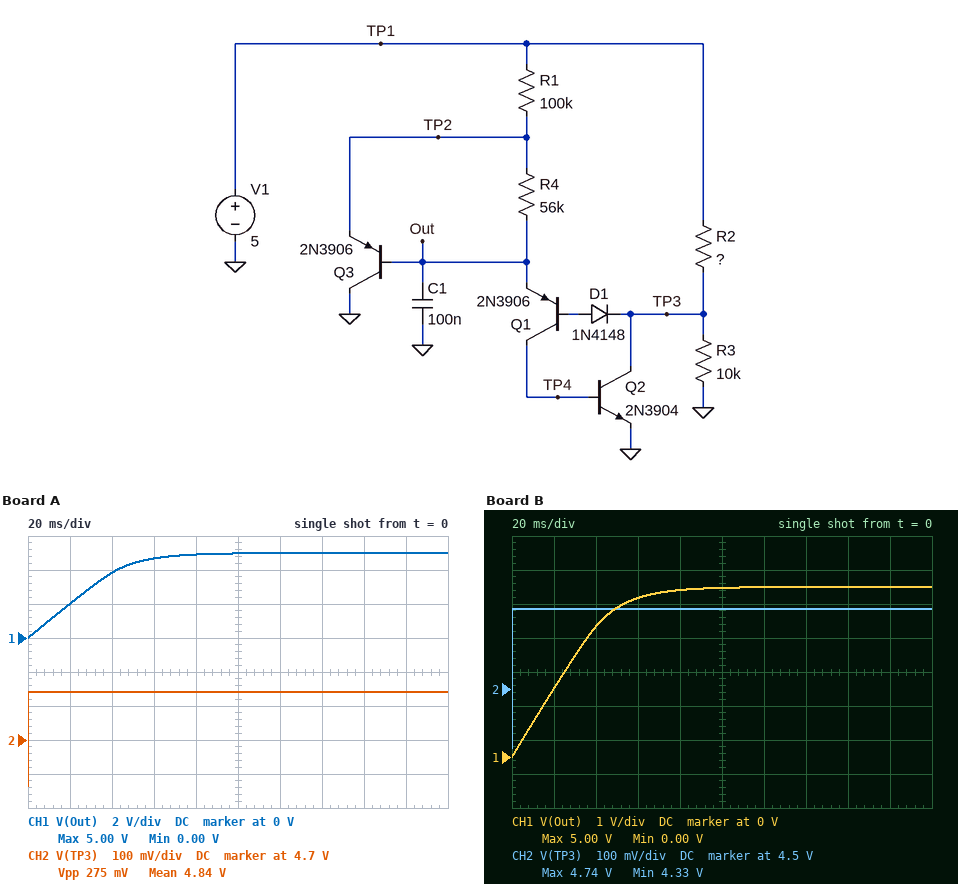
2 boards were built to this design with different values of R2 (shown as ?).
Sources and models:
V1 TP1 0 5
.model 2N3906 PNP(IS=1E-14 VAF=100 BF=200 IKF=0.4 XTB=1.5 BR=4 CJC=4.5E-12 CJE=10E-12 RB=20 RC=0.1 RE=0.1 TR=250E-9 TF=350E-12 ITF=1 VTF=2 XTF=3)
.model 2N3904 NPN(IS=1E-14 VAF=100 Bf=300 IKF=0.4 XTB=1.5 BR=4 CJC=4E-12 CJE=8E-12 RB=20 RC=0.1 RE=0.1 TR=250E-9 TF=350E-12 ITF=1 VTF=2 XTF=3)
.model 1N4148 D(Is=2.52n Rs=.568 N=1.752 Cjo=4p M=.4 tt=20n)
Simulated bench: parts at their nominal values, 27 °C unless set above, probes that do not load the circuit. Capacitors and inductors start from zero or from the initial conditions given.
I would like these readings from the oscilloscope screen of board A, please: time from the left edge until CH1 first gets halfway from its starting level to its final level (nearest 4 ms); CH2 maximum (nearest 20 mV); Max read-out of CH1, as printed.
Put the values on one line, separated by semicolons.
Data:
24 ms; 4.84 V; 5.00 V
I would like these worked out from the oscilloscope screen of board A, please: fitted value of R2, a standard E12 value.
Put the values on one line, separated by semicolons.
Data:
330 Ω
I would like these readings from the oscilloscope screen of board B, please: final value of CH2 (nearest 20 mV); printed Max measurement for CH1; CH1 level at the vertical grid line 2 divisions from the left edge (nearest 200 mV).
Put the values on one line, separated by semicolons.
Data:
4.74 V; 5.00 V; 3.8 V
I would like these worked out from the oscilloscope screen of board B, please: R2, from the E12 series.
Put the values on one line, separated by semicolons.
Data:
560 Ω
